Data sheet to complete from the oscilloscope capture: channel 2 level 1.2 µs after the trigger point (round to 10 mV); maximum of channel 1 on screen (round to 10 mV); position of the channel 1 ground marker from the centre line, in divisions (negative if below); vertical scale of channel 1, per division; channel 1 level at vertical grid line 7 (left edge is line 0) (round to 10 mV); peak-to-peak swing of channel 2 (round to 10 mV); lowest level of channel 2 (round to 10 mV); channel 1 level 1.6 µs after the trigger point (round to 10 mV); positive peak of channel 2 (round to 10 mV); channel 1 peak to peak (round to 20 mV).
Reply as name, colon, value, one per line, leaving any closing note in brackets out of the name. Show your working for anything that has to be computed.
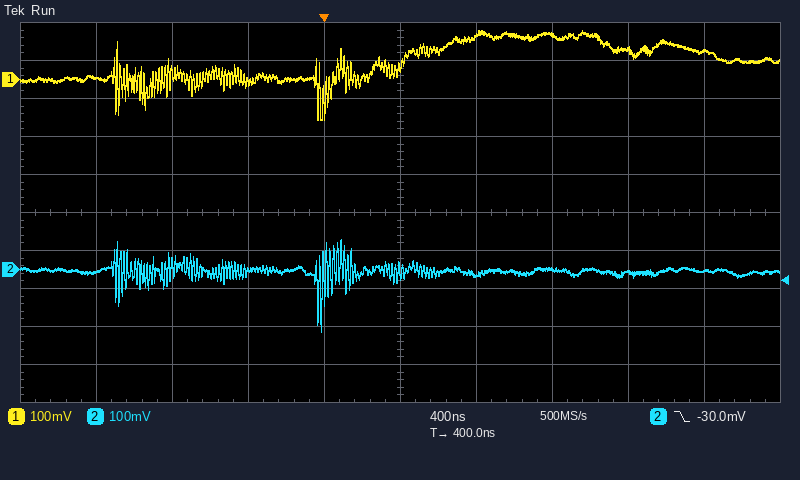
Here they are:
channel 2 level 1.2 µs after the trigger point: 0 mV
maximum of channel 1 on screen: 130 mV
position of the channel 1 ground marker from the centre line, in divisions: +3.5 div
vertical scale of channel 1, per division: 100 mV
channel 1 level at vertical grid line 7 (left edge is line 0): 120 mV
peak-to-peak swing of channel 2: 80 mV − (-160 mV) = 240 mV
lowest level of channel 2: -160 mV
channel 1 level 1.6 µs after the trigger point: 80 mV
positive peak of channel 2: 80 mV
channel 1 peak to peak: 240 mV
